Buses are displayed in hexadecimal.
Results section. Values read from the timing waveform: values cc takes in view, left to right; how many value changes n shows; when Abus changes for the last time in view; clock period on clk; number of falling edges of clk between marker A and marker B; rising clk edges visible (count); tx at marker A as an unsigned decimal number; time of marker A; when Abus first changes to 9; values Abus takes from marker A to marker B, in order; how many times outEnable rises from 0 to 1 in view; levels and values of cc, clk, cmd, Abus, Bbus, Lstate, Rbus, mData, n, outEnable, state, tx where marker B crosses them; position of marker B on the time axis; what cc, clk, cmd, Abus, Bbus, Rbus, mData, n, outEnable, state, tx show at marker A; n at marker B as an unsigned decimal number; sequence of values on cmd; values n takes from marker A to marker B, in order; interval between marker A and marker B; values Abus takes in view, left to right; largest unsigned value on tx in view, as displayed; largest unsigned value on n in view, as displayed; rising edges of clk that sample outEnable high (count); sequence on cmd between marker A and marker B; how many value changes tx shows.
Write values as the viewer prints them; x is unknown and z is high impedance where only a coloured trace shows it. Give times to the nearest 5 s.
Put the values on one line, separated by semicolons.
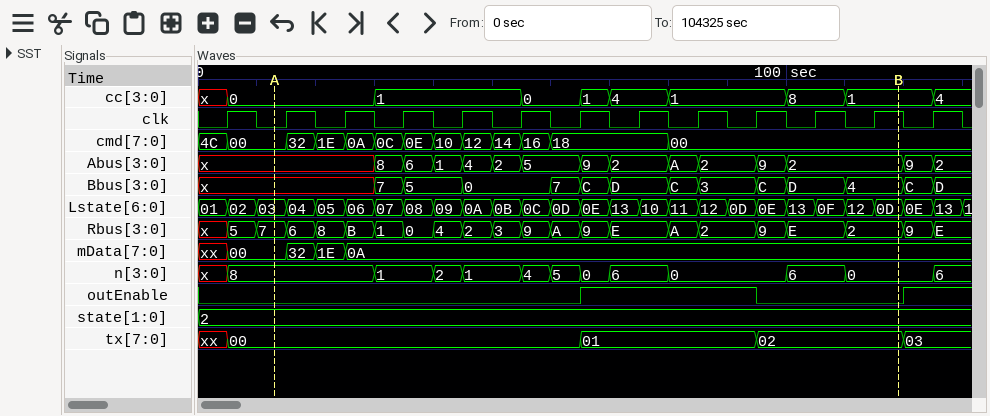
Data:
x, 0, 1, 0, 1, 4, 1, 8, 1, 4; 12; 125 s; 10 s; 10; 13; 0; 15 s; 65 s; x, 8, 6, 1, 4, 2, 5, 9, 2, A, 2, 9, 2; 2; cc=1, clk=1, cmd=00, Abus=2, Bbus=4, Lstate=0D, Rbus=2, mData=0A, n=0, outEnable=0, state=2, tx=02; 120 s; cc=0, clk=0, cmd=00, Abus=x, Bbus=x, Rbus=7, mData=00, n=8, outEnable=0, state=2, tx=00; 0; 4C, 00, 32, 1E, 0A, 0C, 0E, 10, 12, 14, 16, 18, 00; 8, 1, 2, 1, 4, 5, 0, 6, 0, 6, 0; 105 s; x, 8, 6, 1, 4, 2, 5, 9, 2, A, 2, 9, 2, 9, 2; 03; 8; 4; 00, 32, 1E, 0A, 0C, 0E, 10, 12, 14, 16, 18, 00; 4
